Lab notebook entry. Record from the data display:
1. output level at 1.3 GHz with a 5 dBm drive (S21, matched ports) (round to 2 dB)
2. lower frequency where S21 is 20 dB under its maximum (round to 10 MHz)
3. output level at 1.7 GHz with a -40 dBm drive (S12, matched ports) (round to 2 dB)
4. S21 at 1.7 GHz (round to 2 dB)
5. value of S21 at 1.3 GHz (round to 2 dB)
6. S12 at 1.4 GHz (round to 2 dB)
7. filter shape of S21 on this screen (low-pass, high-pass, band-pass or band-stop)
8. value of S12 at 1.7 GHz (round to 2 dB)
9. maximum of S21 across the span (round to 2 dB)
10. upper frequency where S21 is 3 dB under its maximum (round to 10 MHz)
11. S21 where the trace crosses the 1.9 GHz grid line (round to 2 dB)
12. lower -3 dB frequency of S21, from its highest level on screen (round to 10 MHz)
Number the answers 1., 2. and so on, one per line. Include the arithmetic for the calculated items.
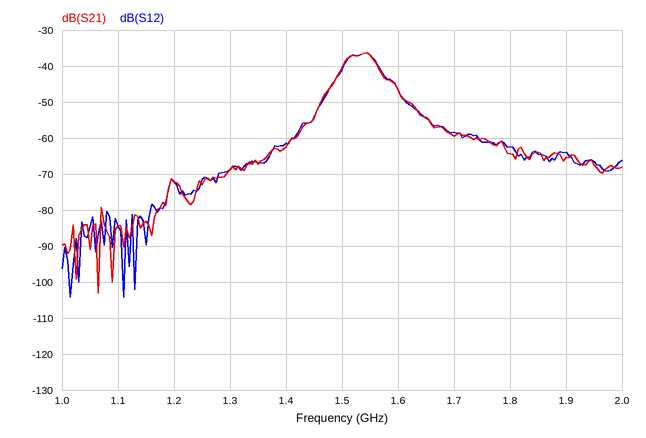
1. 5 dBm + (-68 dB) = -64 dBm
2. 1.43 GHz
3. -40 dBm + (-58 dB) = -98 dBm
4. -60 dB
5. -68 dB
6. -62 dB
7. band-pass
8. -58 dB
9. -36 dB
10. 1.56 GHz
11. -66 dB
12. 1.50 GHz
